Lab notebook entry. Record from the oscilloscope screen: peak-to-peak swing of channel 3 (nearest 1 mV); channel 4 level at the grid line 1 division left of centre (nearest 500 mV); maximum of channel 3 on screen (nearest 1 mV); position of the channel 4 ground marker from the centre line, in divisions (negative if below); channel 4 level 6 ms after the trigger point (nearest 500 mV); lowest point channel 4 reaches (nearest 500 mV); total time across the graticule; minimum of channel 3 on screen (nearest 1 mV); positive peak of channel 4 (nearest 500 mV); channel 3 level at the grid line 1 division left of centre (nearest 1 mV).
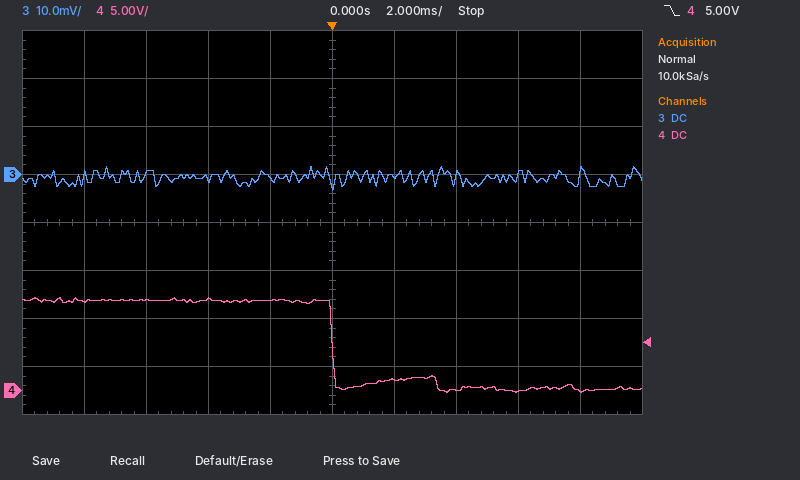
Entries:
5 mV
9.5 V
2 mV
-3.5 div
0.0 V
0.0 V
20 ms
-3 mV
9.5 V
-1 mV
